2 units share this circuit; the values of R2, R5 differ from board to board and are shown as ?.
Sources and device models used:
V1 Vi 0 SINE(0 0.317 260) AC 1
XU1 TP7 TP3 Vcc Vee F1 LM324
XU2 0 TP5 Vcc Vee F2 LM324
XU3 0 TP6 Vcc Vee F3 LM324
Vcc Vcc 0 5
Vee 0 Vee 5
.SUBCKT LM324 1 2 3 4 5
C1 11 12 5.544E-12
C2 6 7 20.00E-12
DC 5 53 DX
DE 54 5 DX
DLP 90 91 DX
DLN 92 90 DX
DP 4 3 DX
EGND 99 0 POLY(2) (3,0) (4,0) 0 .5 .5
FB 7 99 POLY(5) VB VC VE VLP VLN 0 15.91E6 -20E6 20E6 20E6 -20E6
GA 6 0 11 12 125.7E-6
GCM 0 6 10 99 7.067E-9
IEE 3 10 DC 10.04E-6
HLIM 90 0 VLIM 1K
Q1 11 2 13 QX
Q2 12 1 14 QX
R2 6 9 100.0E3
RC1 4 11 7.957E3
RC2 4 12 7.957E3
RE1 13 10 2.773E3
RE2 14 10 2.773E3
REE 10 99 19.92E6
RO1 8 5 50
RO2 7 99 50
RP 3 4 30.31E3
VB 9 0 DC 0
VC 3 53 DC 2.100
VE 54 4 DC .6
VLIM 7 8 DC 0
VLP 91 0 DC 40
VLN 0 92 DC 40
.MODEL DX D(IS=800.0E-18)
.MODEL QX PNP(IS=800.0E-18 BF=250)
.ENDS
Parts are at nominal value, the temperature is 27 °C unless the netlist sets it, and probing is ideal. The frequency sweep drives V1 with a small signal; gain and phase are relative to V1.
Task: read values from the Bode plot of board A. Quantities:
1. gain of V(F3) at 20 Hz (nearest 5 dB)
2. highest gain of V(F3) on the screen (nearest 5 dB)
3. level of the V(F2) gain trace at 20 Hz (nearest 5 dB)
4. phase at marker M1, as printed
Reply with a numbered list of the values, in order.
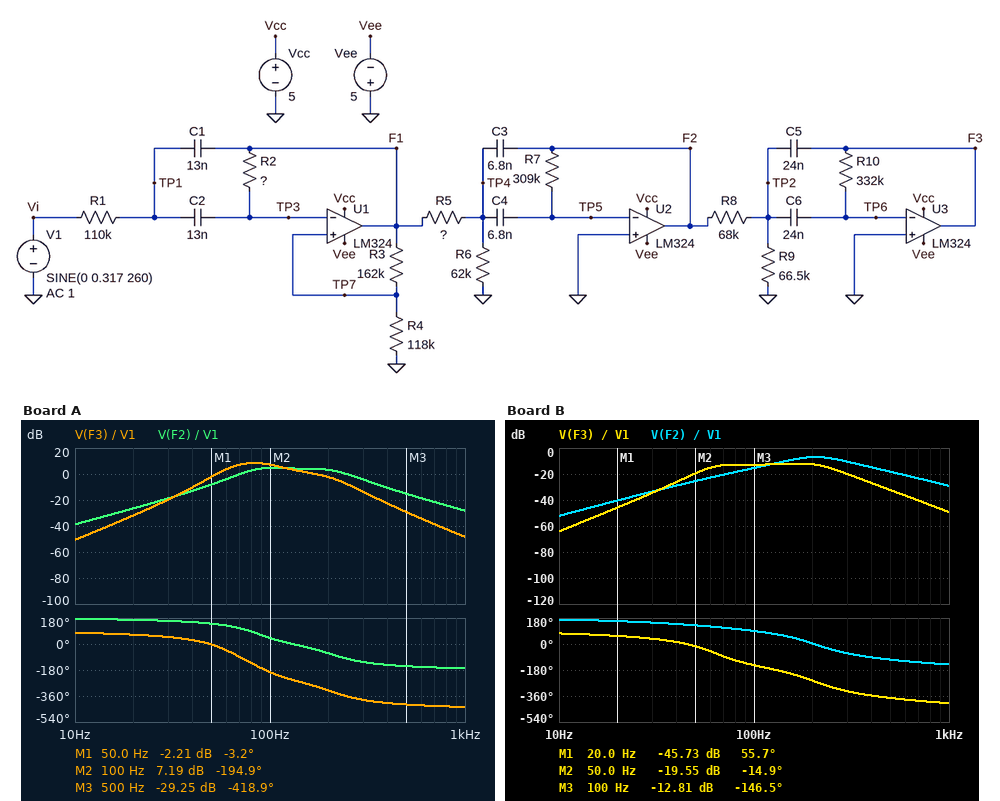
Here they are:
1. -30 dB
2. 10 dB
3. -25 dB
4. -3.2 deg
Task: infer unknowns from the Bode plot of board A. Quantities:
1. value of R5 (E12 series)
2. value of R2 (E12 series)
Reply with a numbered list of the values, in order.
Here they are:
1. 120 kΩ
2. 180 kΩ
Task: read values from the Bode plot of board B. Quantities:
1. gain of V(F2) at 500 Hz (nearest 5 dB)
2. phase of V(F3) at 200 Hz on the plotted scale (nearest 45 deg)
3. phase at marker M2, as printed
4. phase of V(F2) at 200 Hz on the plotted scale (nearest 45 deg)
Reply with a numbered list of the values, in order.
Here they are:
1. -20 dB
2. -270 deg
3. -14.9 deg
4. 0 deg
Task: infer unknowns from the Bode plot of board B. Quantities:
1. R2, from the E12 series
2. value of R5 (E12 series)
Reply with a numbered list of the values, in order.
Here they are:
1. 39 kΩ
2. 120 kΩ
